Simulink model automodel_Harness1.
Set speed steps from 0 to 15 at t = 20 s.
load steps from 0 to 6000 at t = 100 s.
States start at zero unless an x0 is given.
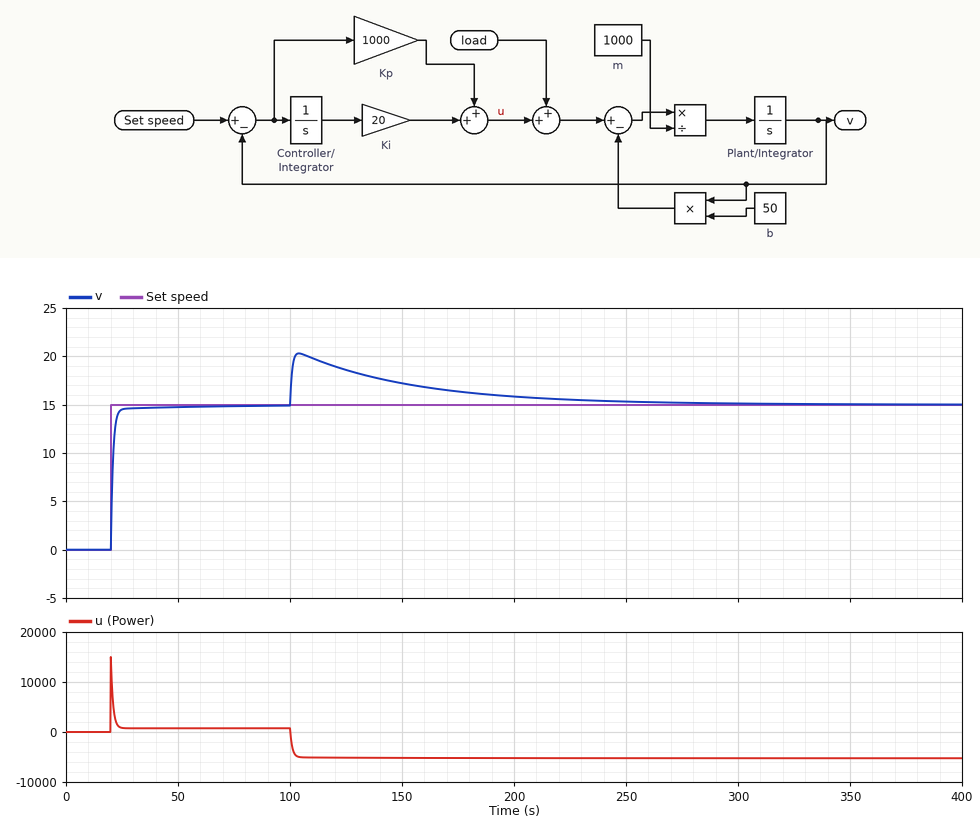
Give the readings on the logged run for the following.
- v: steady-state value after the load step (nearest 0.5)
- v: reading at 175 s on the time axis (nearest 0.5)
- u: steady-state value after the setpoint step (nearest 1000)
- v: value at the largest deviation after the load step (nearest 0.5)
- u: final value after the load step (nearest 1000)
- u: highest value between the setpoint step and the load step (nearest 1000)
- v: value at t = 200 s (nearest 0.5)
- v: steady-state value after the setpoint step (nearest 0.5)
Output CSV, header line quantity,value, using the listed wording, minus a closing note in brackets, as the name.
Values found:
quantity,value
v: steady-state value after the load step,15.0
v: reading at 175 s on the time axis,16.5
u: steady-state value after the setpoint step,1000
v: value at the largest deviation after the load step,20.5
u: final value after the load step,-5000
u: highest value between the setpoint step and the load step,15000
v: value at t = 200 s,16.0
v: steady-state value after the setpoint step,15.0
